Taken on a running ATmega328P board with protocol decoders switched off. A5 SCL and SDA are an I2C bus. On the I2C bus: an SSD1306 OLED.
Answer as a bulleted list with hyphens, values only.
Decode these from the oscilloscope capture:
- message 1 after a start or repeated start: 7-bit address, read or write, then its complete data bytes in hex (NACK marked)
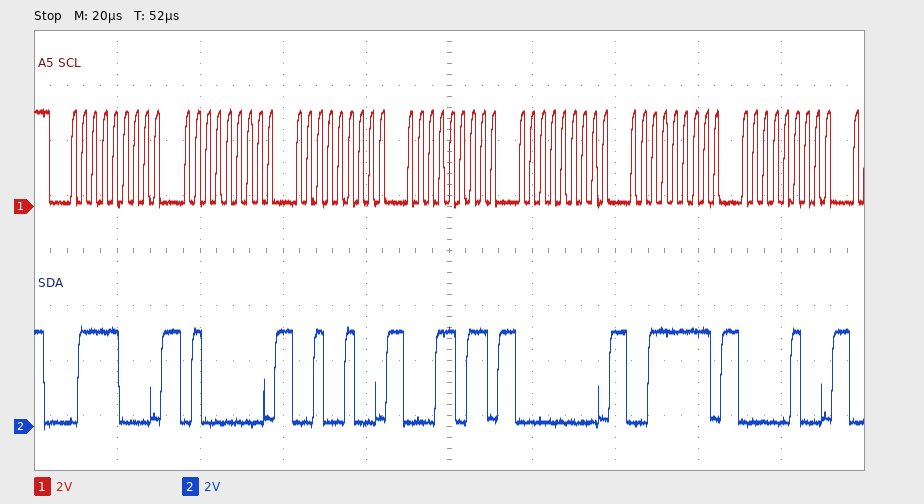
- 0x3C write: 40 24 1B 00 3F 04
